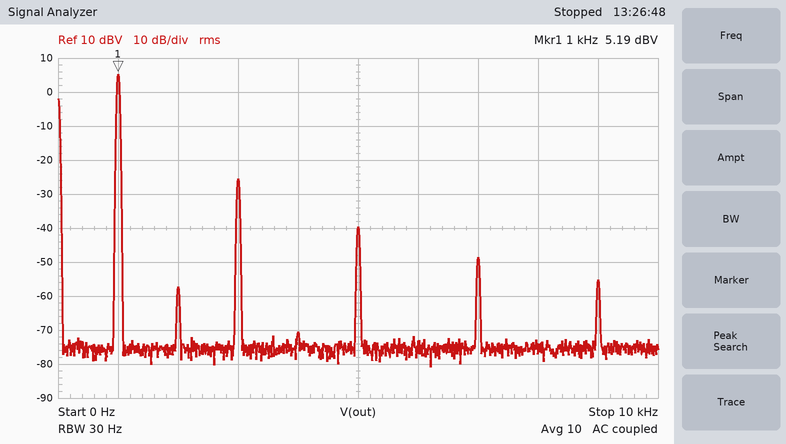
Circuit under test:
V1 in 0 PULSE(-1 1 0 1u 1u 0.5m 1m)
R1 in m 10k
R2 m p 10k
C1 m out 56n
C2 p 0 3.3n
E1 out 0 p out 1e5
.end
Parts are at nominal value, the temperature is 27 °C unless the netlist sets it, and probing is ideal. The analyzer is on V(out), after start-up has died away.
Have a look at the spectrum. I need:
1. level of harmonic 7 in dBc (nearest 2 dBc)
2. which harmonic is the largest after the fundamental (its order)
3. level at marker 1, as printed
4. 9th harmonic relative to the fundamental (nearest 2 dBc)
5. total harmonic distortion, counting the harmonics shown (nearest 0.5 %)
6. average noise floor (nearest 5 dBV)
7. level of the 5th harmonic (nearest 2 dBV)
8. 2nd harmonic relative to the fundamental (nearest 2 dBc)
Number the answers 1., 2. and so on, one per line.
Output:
1. -54 dBc
2. 3
3. 5.19 dBV
4. -60 dBc
5. 3.0 %
6. -75 dBV
7. -40 dBV
8. -62 dBc
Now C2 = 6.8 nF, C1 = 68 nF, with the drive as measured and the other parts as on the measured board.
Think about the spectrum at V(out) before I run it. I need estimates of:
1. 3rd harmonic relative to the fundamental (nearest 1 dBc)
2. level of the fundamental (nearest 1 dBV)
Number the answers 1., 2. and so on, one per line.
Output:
1. -32 dBc
2. -2 dBV
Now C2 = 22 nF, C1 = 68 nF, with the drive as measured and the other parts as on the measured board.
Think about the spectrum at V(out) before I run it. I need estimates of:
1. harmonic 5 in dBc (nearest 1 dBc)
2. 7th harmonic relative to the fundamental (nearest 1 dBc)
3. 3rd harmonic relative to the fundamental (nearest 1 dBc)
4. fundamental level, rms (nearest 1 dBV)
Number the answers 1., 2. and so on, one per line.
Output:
1. -42 dBc
2. -51 dBc
3. -29 dBc
4. -16 dBV
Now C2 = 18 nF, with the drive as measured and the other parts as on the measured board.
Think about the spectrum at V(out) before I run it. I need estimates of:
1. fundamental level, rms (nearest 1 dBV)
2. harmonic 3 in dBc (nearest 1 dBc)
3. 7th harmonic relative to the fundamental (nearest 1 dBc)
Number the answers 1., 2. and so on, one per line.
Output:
1. -12 dBV
2. -29 dBc
3. -51 dBc
